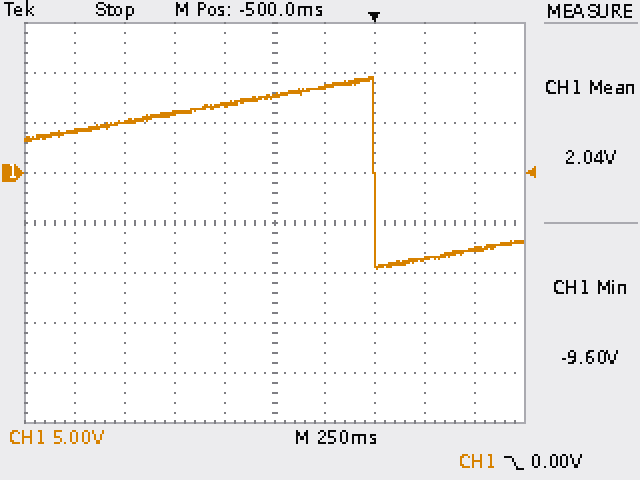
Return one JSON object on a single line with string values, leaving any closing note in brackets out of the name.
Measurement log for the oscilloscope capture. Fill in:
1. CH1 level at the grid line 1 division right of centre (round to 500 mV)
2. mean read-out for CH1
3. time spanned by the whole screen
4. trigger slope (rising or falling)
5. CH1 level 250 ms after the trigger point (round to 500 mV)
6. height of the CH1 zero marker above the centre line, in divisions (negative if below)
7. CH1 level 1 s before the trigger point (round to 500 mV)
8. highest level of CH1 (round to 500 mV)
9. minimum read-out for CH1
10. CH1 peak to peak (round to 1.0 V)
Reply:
{"CH1 level at the grid line 1 division right of centre": "8.5 V", "mean read-out for CH1": "2.04 V", "time spanned by the whole screen": "2.5 s", "trigger slope": "falling", "CH1 level 250 ms after the trigger point": "-8.5 V", "height of the CH1 zero marker above the centre line, in divisions": "+1.0 div", "CH1 level 1 s before the trigger point": "6.0 V", "highest level of CH1": "9.5 V", "minimum read-out for CH1": "-9.60 V", "CH1 peak to peak": "19.0 V"}
